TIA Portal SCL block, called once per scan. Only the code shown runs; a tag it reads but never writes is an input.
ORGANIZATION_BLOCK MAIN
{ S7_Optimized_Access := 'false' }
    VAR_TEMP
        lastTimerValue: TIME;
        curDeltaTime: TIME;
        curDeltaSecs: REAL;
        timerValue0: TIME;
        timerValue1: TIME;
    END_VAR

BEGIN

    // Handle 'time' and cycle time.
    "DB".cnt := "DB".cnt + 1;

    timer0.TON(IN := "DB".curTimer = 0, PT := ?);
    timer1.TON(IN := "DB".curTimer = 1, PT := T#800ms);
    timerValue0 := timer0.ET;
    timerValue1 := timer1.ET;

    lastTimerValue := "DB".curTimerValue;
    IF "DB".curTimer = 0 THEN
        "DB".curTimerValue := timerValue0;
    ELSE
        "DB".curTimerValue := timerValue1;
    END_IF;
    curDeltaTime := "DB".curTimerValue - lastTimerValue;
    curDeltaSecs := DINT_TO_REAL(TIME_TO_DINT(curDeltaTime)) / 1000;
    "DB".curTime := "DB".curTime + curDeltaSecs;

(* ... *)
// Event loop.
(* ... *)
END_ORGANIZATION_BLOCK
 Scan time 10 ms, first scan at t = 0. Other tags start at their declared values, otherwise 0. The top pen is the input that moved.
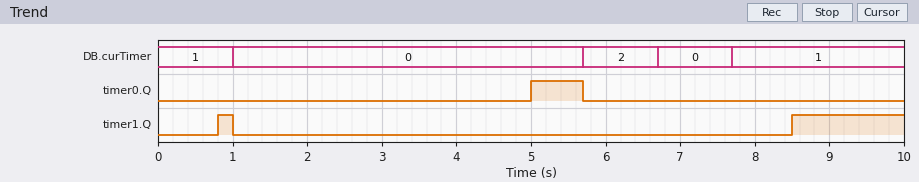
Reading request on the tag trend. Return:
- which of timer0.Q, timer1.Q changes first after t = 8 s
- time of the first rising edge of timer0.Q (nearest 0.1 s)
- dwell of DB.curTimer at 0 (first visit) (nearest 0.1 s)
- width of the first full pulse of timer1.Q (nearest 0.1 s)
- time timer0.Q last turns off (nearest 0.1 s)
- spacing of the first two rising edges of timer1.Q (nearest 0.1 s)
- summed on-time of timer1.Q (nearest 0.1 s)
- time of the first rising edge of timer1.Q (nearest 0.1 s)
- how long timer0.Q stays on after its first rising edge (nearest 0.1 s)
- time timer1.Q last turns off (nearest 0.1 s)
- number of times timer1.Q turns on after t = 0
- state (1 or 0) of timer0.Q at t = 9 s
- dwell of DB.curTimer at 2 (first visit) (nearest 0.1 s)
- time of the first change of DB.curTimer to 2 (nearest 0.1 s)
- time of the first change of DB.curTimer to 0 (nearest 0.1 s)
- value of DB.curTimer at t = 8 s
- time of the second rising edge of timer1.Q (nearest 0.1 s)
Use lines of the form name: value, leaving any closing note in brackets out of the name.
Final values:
which of timer0.Q, timer1.Q changes first after t = 8 s: timer1.Q
time of the first rising edge of timer0.Q: 5.0 s
dwell of DB.curTimer at 0 (first visit): 4.7 s
width of the first full pulse of timer1.Q: 0.2 s
time timer0.Q last turns off: 5.7 s
spacing of the first two rising edges of timer1.Q: 7.7 s
summed on-time of timer1.Q: 1.7 s
time of the first rising edge of timer1.Q: 0.8 s
how long timer0.Q stays on after its first rising edge: 0.7 s
time timer1.Q last turns off: 1.0 s
number of times timer1.Q turns on after t = 0: 2
state (1 or 0) of timer0.Q at t = 9 s: 0
dwell of DB.curTimer at 2 (first visit): 1.0 s
time of the first change of DB.curTimer to 2: 5.7 s
time of the first change of DB.curTimer to 0: 1.0 s
value of DB.curTimer at t = 8 s: 1
time of the second rising edge of timer1.Q: 8.5 s
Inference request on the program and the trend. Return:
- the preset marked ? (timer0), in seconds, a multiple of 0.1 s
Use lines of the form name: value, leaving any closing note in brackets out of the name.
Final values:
the preset marked ? (timer0), in seconds, a multiple of 0.1 s: 4.0 s
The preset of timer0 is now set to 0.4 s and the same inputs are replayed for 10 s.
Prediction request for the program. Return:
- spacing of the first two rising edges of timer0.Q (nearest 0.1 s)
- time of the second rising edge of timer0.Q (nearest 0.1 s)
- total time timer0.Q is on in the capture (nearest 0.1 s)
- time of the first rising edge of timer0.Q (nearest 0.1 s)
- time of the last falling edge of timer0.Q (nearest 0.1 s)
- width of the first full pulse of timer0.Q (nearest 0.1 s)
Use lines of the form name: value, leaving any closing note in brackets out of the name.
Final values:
spacing of the first two rising edges of timer0.Q: 5.7 s
time of the second rising edge of timer0.Q: 7.1 s
total time timer0.Q is on in the capture: 4.9 s
time of the first rising edge of timer0.Q: 1.4 s
time of the last falling edge of timer0.Q: 7.7 s
width of the first full pulse of timer0.Q: 4.3 s
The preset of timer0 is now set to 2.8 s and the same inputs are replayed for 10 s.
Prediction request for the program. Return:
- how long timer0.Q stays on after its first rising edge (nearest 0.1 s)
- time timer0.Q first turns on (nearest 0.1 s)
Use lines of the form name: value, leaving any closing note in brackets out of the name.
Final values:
how long timer0.Q stays on after its first rising edge: 1.9 s
time timer0.Q first turns on: 3.8 s
